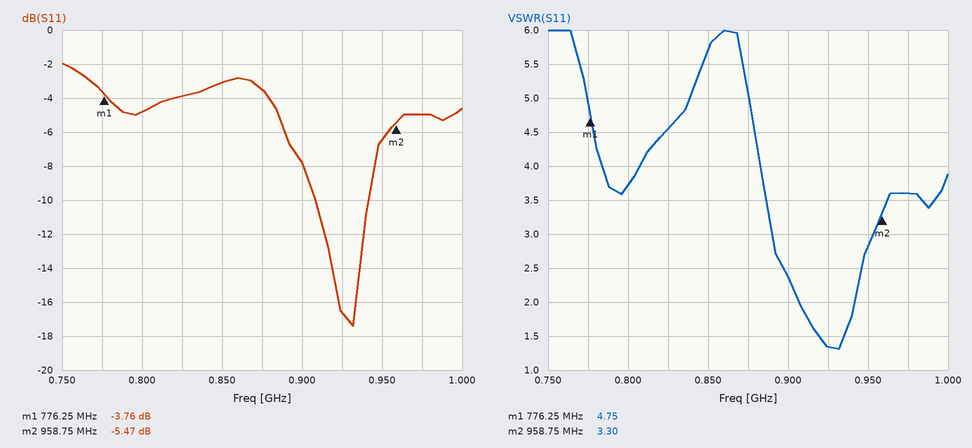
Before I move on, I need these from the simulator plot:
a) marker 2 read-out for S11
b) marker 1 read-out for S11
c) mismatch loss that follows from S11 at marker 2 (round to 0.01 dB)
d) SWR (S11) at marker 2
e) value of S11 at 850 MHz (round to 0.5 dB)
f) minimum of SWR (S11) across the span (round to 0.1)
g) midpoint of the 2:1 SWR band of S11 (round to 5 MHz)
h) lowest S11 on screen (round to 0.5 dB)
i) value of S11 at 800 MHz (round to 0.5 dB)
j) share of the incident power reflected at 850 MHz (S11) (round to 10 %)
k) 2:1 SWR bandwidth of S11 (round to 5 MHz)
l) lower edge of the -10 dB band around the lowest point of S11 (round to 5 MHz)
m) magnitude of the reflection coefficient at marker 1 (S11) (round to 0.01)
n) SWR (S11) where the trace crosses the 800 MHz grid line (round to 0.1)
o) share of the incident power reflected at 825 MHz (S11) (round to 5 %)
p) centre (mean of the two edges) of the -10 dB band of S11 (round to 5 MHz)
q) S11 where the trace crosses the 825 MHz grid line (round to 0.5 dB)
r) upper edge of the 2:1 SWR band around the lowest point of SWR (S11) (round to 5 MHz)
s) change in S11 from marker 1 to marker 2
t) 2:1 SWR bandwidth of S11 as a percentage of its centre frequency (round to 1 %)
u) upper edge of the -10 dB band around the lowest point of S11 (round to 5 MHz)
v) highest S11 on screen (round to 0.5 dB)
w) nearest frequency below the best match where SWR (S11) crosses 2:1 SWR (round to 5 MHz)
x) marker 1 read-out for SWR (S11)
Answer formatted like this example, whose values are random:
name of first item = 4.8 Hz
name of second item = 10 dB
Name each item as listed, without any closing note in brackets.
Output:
marker 2 read-out for S11 = -5.47 dB
marker 1 read-out for S11 = -3.76 dB
mismatch loss that follows from S11 at marker 2 = 1.45 dB
SWR (S11) at marker 2 = 3.30
value of S11 at 850 MHz = -3.0 dB
minimum of SWR (S11) across the span = 1.3
midpoint of the 2:1 SWR band of S11 = 925 MHz
lowest S11 on screen = -17.5 dB
value of S11 at 800 MHz = -5.0 dB
share of the incident power reflected at 850 MHz (S11) = 50 %
2:1 SWR bandwidth of S11 = 35 MHz
lower edge of the -10 dB band around the lowest point of S11 = 910 MHz
magnitude of the reflection coefficient at marker 1 (S11) = 0.65
SWR (S11) where the trace crosses the 800 MHz grid line = 3.7
share of the incident power reflected at 825 MHz (S11) = 40 %
centre (mean of the two edges) of the -10 dB band of S11 = 925 MHz
S11 where the trace crosses the 825 MHz grid line = -4.0 dB
upper edge of the 2:1 SWR band around the lowest point of SWR (S11) = 940 MHz
change in S11 from marker 1 to marker 2 = -1.71 dB
2:1 SWR bandwidth of S11 as a percentage of its centre frequency = 4 %
upper edge of the -10 dB band around the lowest point of S11 = 940 MHz
highest S11 on screen = -2.0 dB
nearest frequency below the best match where SWR (S11) crosses 2:1 SWR = 905 MHz
marker 1 read-out for SWR = 4.75
